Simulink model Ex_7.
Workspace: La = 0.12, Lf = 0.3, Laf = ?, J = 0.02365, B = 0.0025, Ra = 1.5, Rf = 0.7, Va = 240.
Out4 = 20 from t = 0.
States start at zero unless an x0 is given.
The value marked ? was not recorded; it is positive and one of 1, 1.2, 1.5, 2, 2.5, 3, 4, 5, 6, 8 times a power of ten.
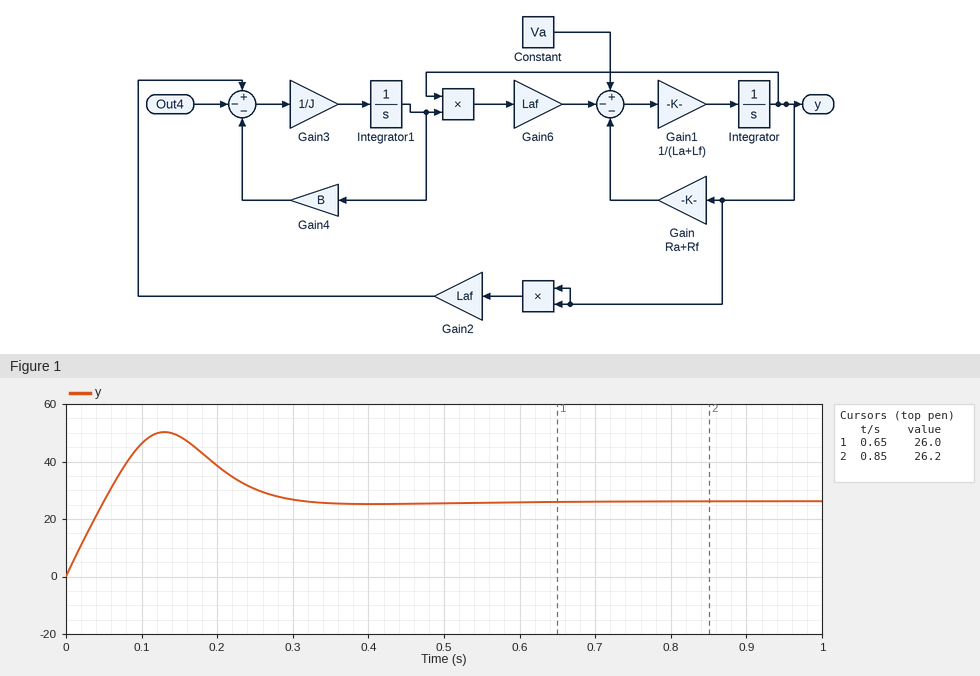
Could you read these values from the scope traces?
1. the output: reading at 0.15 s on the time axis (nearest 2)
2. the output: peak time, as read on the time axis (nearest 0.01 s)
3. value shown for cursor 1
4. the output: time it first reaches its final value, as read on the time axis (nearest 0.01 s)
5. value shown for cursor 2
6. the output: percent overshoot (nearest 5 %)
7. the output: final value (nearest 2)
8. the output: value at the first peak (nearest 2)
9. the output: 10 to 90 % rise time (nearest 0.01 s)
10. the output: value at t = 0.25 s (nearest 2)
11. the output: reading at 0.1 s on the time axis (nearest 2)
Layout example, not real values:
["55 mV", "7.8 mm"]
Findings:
["48", "0.13 s", "26.0", "0.05 s", "26.2", "90 %", "26", "50", "0.04 s", "30", "46"]
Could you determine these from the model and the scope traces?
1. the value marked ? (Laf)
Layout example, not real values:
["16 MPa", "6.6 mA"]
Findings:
["0.03"]
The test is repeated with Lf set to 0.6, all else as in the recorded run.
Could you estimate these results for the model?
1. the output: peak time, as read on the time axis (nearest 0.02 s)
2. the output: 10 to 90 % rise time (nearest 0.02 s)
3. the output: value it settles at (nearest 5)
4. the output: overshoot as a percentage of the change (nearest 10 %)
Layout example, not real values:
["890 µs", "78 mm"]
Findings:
["0.20 s", "0.06 s", "25", "80 %"]
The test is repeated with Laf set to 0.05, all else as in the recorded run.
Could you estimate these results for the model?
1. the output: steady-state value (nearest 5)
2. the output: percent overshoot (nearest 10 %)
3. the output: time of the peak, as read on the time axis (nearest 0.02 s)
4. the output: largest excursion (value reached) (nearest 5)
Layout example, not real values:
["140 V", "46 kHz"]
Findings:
["20", "100 %", "0.10 s", "40"]
